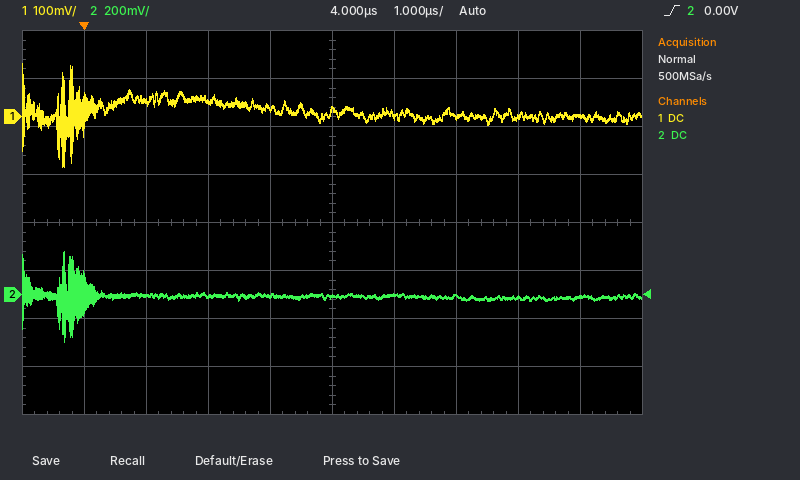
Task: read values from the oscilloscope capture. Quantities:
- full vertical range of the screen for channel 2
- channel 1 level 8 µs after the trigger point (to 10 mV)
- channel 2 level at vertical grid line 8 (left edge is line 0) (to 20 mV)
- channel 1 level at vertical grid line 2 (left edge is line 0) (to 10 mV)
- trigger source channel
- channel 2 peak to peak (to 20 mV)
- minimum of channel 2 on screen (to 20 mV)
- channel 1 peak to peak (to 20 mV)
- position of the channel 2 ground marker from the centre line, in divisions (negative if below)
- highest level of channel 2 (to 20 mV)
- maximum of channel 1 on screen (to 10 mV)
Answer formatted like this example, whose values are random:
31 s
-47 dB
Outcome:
1.6 V
0 mV
-20 mV
30 mV
channel 2
380 mV
-200 mV
220 mV
-1.5 div
180 mV
110 mV
